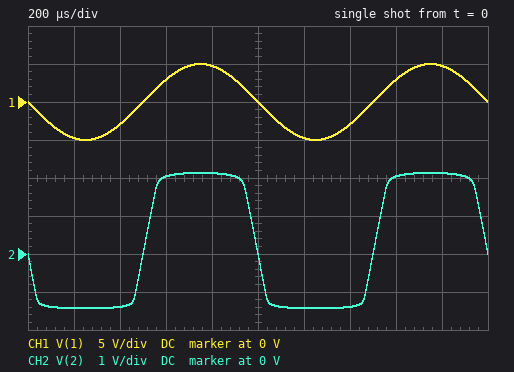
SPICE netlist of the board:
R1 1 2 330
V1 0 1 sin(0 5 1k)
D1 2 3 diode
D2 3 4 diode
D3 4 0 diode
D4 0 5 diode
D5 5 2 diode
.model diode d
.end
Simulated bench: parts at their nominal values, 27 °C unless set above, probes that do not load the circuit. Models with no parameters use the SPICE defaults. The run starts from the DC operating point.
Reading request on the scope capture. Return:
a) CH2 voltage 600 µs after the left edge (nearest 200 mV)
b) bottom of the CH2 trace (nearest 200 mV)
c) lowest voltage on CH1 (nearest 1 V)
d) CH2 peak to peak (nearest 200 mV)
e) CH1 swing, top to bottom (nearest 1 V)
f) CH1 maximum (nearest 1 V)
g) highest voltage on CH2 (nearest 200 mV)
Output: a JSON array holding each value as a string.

["2.0 V", "-1.4 V", "-5 V", "3.6 V", "10 V", "5 V", "2.2 V"]
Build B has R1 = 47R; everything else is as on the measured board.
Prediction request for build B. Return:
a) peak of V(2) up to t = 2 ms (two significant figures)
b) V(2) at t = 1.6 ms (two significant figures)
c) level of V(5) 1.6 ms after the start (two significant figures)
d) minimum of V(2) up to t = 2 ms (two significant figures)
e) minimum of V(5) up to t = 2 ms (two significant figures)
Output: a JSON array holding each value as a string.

["2.3 V", "2.2 V", "1.1 V", "-1.5 V", "-770 mV"]
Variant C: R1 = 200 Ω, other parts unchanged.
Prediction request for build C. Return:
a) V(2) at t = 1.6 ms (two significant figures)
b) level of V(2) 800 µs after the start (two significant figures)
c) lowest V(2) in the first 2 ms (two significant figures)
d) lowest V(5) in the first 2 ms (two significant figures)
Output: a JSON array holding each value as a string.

["2.1 V", "2.2 V", "-1.5 V", "-730 mV"]
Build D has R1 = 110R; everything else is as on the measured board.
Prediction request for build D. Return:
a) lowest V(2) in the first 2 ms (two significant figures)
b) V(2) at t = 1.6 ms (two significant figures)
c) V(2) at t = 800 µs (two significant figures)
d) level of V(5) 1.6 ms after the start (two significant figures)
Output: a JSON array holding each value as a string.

["-1.5 V", "2.1 V", "2.2 V", "1.1 V"]
